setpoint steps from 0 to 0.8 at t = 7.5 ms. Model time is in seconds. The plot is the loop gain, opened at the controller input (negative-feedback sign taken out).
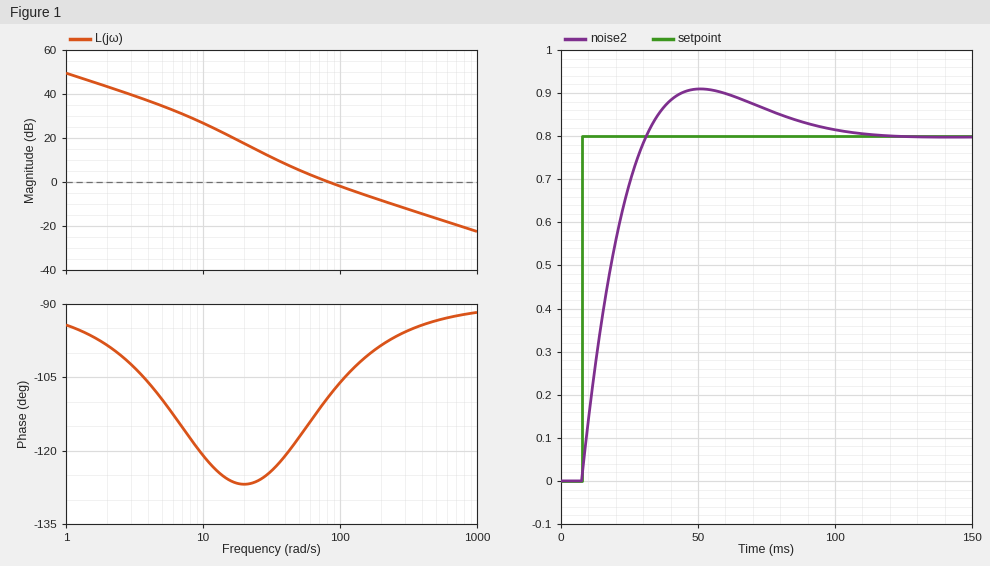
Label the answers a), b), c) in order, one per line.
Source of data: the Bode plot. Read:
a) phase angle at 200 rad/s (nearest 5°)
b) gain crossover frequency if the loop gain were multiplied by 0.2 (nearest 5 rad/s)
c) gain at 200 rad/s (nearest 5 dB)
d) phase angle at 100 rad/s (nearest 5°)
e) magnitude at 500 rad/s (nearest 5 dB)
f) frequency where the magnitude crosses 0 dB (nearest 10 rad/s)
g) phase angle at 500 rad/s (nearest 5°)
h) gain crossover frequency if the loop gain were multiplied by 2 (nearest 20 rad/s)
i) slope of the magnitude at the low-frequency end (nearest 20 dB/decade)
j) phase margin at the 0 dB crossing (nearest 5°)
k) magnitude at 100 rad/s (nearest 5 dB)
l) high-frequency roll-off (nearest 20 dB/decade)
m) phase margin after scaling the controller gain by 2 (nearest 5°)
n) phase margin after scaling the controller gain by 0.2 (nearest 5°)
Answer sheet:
a) -100°
b) 25 rad/s
c) -10 dB
d) -105°
e) -15 dB
f) 80 rad/s
g) -95°
h) 160 rad/s
i) -20 dB/decade
j) 70°
k) 0 dB
l) -20 dB/decade
m) 80°
n) 55°
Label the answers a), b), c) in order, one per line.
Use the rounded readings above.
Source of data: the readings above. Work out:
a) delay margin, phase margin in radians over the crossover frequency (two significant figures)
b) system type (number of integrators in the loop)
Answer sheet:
a) 0.015 s
b) 1
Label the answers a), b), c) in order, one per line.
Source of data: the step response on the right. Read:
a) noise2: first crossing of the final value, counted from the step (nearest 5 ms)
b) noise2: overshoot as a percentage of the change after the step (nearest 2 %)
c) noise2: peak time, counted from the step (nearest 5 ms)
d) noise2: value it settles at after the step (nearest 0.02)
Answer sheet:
a) 25 ms
b) 14 %
c) 45 ms
d) 0.80
